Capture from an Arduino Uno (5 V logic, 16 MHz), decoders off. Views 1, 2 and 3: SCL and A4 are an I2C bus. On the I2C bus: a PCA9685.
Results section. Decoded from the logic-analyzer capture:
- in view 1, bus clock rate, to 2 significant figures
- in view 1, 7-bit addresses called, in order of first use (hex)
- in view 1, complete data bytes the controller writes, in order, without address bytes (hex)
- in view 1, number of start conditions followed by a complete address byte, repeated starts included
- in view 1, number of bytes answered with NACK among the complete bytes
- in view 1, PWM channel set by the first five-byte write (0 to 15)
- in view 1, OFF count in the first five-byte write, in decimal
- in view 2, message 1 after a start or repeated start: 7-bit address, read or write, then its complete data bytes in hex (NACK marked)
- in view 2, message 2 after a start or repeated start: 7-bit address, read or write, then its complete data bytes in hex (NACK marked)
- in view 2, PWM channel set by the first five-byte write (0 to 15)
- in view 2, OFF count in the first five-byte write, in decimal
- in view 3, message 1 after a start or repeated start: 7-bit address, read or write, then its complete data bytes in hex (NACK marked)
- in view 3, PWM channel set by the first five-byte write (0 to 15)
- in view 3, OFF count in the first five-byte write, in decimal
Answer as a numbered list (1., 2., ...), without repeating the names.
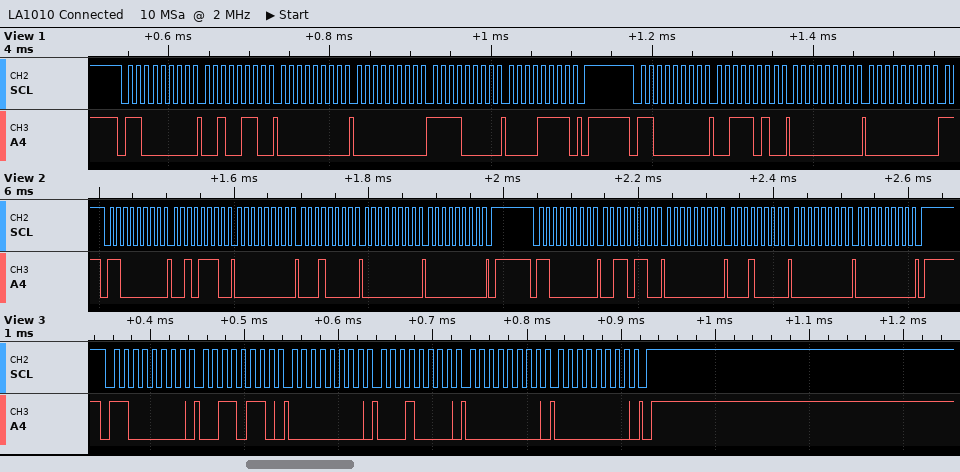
1. 100 kHz
2. 0x60
3. 26 00 00 F0 0F 3A 00 00
4. 2
5. 0
6. 8
7. 4080
8. 0x60 write: 2E 00 10 00 00
9. 0x60 write: 36 00 10 00 00
10. 10
11. 0
12. 0x60 write: 36 00 10 00 00
13. 12
14. 0
